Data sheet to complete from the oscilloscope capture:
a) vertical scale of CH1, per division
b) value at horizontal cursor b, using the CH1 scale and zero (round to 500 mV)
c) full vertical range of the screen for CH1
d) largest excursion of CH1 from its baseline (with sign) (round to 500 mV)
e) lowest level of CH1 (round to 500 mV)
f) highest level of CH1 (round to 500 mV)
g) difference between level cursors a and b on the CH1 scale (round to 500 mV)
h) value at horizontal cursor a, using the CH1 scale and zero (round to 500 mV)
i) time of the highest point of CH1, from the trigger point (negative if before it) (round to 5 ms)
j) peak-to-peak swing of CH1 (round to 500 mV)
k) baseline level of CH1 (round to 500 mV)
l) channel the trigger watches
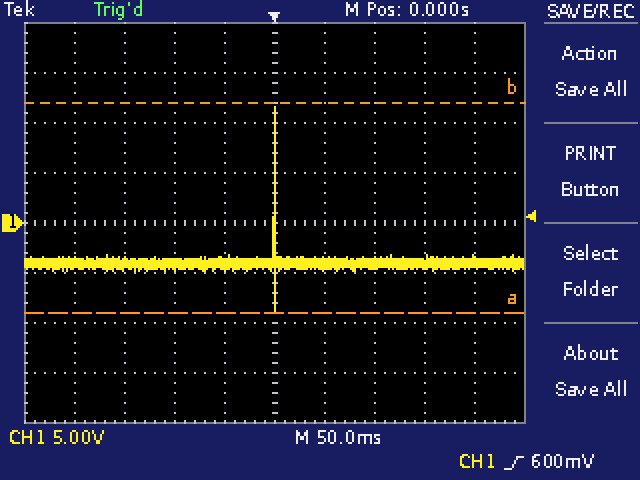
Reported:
5 V
12.0 V
40 V
+15.5 V
-9.0 V
11.5 V
21.0 V
-9.0 V
0 ms
20.5 V
-4.0 V
CH1
